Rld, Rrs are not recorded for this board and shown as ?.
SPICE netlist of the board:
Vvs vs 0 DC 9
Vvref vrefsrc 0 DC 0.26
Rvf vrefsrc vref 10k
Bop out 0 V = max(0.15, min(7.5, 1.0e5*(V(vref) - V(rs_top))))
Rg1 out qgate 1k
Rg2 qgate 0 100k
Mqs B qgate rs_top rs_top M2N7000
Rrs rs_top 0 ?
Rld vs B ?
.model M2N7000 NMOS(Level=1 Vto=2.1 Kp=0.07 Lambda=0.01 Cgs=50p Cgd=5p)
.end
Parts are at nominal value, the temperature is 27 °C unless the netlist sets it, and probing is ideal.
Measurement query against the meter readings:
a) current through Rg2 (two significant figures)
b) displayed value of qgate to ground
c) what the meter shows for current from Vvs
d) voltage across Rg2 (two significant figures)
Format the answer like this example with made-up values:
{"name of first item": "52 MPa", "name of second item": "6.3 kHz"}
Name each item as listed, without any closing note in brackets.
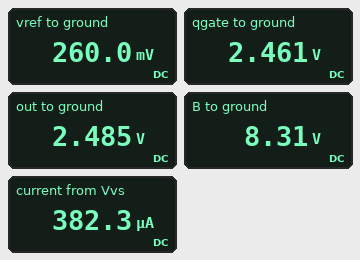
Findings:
{"current through Rg2": "25 µA", "displayed value of qgate to ground": "2.461 V", "what the meter shows for current from Vvs": "382.3 µA", "voltage across Rg2": "2.5 V"}
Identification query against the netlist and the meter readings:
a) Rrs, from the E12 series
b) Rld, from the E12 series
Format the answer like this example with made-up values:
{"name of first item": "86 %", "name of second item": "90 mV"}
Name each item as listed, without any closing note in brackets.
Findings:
{"Rrs, from the E12 series": "680 Ω", "Rld, from the E12 series": "1.8 kΩ"}
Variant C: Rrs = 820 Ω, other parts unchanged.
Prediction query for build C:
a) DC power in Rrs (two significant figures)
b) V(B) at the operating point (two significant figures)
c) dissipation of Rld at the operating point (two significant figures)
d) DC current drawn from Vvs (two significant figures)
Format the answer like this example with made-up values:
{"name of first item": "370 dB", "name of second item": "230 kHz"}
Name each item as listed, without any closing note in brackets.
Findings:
{"DC power in Rrs": "82 µW", "V(B) at the operating point": "8.4 V", "dissipation of Rld at the operating point": "180 µW", "DC current drawn from Vvs": "320 µA"}
